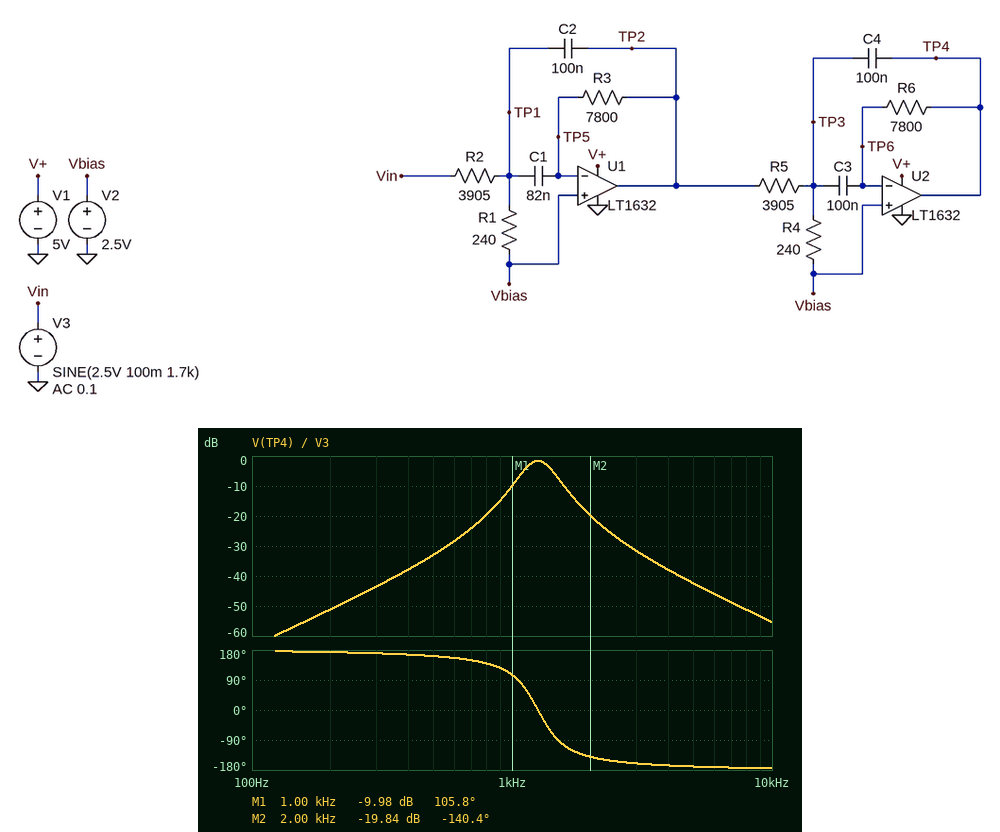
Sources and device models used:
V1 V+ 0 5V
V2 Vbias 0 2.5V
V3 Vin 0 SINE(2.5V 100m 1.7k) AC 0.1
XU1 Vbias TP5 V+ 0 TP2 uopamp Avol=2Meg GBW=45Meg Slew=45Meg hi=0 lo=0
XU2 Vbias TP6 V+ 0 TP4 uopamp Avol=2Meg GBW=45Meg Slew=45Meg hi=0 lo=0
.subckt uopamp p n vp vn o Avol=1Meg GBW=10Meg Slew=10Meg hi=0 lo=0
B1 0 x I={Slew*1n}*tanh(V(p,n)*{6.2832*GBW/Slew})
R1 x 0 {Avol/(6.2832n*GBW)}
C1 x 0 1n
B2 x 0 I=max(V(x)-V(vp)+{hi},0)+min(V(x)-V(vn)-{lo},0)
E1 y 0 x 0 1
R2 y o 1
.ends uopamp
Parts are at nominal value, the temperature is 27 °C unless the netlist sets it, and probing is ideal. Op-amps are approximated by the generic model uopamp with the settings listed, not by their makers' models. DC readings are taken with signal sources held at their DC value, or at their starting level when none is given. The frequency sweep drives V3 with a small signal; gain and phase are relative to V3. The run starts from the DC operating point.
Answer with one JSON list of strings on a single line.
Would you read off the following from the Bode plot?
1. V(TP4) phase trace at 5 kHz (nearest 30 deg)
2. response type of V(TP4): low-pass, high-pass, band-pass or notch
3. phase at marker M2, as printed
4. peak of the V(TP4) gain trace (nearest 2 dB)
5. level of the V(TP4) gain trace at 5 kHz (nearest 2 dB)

["-180 deg", "band-pass", "-140.4 deg", "-2 dB", "-42 dB"]
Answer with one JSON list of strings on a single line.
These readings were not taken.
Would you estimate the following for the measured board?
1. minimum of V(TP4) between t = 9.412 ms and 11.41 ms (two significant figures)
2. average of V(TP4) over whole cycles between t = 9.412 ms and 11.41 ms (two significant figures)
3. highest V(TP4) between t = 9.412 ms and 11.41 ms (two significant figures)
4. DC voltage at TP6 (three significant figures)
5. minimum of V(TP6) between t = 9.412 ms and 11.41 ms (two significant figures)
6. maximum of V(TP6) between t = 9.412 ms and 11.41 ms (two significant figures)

["2.5 V", "2.5 V", "2.5 V", "2.50 V", "2.5 V", "2.5 V"]
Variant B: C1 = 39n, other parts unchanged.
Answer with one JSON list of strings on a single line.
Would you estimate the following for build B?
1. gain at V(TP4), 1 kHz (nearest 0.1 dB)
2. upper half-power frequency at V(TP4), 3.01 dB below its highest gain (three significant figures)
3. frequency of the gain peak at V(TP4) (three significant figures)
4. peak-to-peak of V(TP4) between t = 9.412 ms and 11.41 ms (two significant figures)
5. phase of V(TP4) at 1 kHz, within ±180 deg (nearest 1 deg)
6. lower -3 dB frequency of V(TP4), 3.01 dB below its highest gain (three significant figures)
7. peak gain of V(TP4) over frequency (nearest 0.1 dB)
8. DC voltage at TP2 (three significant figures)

["-20.0 dB", "2.05 kHz", "1.29 kHz", "41 mV", "122 deg", "1.10 kHz", "-13.3 dB", "2.50 V"]
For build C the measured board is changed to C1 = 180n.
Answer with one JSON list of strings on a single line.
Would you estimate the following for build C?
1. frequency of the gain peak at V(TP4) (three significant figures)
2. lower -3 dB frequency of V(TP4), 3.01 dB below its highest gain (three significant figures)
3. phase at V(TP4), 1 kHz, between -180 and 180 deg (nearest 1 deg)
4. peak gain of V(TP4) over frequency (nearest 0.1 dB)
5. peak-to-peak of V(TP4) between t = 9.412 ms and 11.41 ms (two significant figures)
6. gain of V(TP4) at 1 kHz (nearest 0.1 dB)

["1.05 kHz", "845 Hz", "14 deg", "-2.5 dB", "28 mV", "-2.6 dB"]
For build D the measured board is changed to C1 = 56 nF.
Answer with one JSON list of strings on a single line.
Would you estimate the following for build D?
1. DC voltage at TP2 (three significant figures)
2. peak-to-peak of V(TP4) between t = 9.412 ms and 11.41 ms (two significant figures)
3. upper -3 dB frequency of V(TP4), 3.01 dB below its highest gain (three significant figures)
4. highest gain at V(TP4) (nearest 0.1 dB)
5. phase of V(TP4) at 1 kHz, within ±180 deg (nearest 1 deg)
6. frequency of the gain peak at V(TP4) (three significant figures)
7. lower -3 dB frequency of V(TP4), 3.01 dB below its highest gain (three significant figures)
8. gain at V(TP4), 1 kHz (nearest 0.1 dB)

["2.50 V", "58 mV", "1.69 kHz", "-7.5 dB", "117 deg", "1.36 kHz", "1.13 kHz", "-15.5 dB"]
